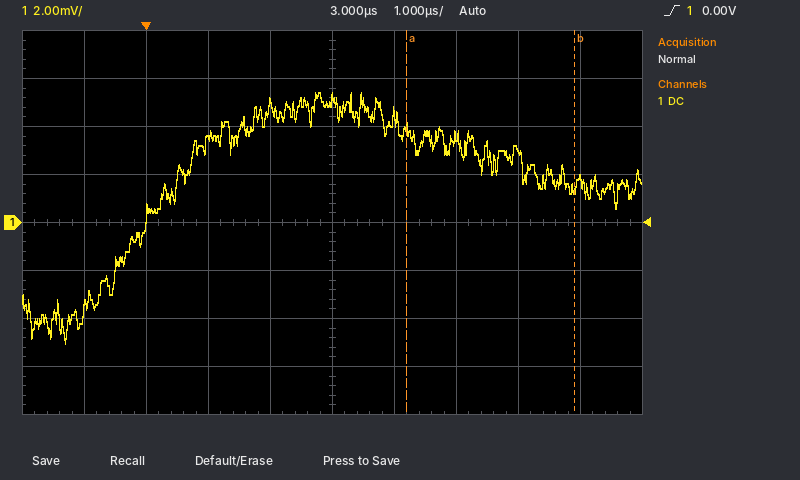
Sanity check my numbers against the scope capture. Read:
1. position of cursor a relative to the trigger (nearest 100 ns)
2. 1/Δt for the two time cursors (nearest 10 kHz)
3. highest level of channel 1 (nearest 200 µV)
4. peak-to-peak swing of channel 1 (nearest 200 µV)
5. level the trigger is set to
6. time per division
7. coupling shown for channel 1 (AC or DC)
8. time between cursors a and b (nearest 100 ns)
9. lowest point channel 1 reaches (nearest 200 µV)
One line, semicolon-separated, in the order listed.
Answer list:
+4.2 µs; 370 kHz; 5.4 mV; 10.4 mV; 0.00 V; 1 µs; DC; 2.7 µs; -5.0 mV
